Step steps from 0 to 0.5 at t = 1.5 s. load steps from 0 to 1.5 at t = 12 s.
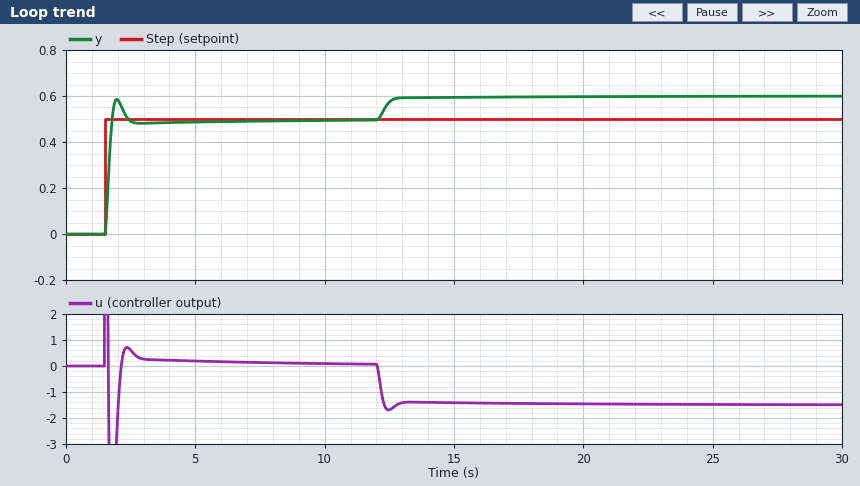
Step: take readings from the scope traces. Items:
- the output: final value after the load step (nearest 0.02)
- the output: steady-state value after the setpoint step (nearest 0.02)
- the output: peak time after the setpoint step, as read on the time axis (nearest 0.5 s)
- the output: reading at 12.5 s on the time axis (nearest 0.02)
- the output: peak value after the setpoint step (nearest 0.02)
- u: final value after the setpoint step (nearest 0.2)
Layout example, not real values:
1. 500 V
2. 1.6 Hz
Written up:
1. 0.60
2. 0.50
3. 2.0 s
4. 0.58
5. 0.58
6. 0.0
